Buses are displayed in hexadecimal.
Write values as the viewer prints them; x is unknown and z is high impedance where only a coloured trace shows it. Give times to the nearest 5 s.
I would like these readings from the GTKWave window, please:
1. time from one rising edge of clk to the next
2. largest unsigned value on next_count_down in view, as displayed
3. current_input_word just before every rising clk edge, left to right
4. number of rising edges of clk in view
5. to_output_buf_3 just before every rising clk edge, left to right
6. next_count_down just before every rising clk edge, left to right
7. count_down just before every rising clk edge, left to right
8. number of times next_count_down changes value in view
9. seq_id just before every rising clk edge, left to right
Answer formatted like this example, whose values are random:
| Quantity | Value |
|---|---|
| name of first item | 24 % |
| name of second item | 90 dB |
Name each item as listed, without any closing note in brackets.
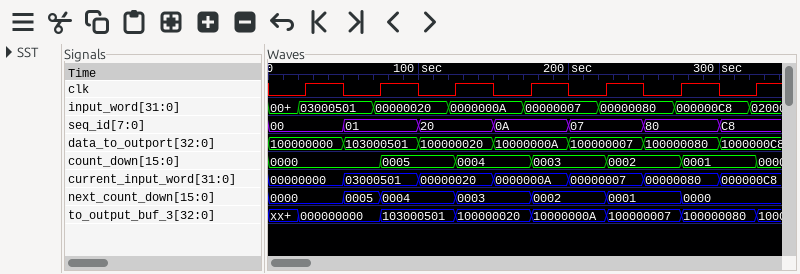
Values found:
| Quantity | Value |
|---|---|
| time from one rising edge of clk to the next | 50 s |
| largest unsigned value on next_count_down in view, as displayed | 0005 |
| current_input_word just before every rising clk edge, left to right | 00000000, 03000501, 00000020, 0000000A, 00000007, 00000080, 000000C8 |
| number of rising edges of clk in view | 7 |
| to_output_buf_3 just before every rising clk edge, left to right | 000000000, 000000000, 103000501, 100000020, 10000000A, 100000007, 100000080 |
| next_count_down just before every rising clk edge, left to right | 0000, 0005, 0004, 0003, 0002, 0001, 0000 |
| count_down just before every rising clk edge, left to right | 0000, 0000, 0005, 0004, 0003, 0002, 0001 |
| number of times next_count_down changes value in view | 6 |
| seq_id just before every rising clk edge, left to right | 00, 01, 20, 0A, 07, 80, C8 |
